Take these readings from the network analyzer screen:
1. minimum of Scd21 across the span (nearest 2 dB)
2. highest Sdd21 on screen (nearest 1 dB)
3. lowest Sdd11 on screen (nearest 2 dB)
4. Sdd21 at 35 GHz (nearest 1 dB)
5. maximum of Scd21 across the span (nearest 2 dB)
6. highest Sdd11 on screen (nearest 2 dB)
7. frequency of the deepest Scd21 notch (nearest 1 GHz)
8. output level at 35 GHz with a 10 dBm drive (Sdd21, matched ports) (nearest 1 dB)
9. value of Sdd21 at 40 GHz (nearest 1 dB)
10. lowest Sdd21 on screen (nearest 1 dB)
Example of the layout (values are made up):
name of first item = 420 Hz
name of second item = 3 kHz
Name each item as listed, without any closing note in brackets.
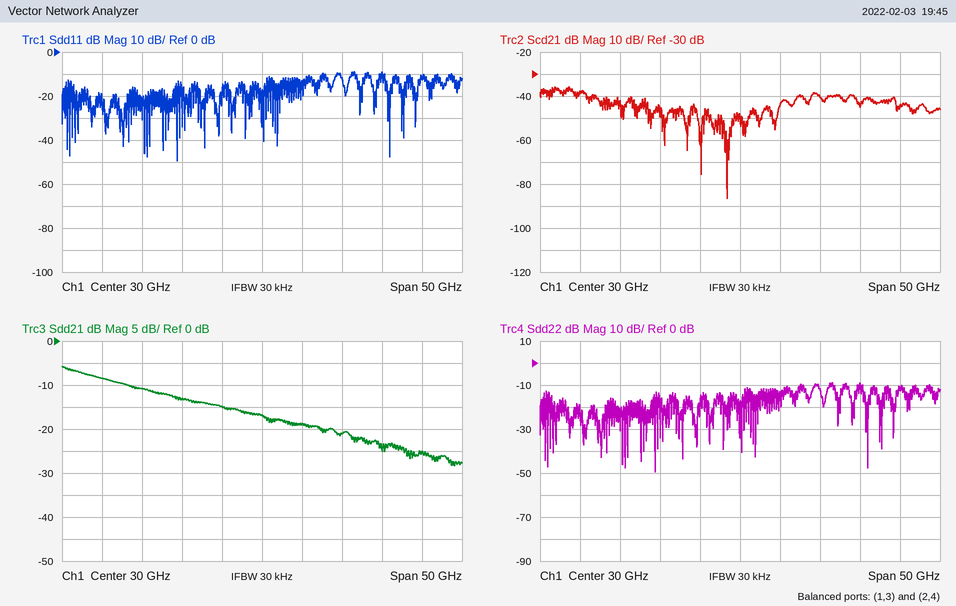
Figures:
minimum of Scd21 across the span = -86 dB
highest Sdd21 on screen = -6 dB
lowest Sdd11 on screen = -50 dB
Sdd21 at 35 GHz = -19 dB
maximum of Scd21 across the span = -36 dB
highest Sdd11 on screen = -8 dB
frequency of the deepest Scd21 notch = 28 GHz
output level at 35 GHz with a 10 dBm drive (Sdd21, matched ports) = -9 dBm
value of Sdd21 at 40 GHz = -21 dB
lowest Sdd21 on screen = -28 dB
